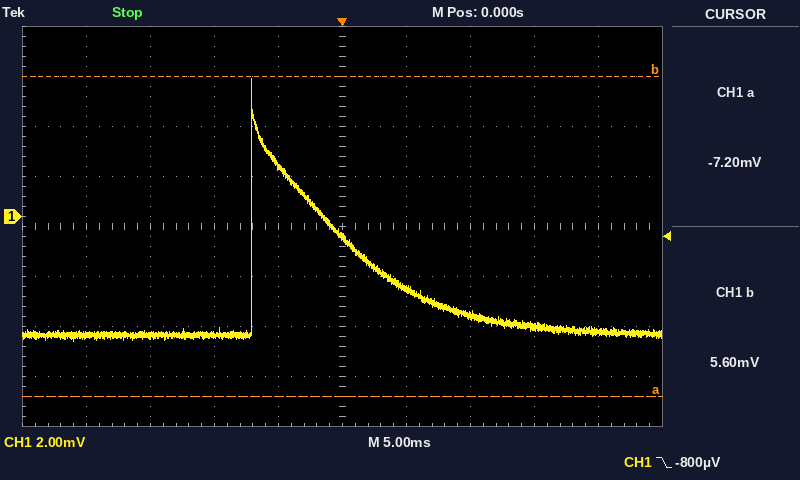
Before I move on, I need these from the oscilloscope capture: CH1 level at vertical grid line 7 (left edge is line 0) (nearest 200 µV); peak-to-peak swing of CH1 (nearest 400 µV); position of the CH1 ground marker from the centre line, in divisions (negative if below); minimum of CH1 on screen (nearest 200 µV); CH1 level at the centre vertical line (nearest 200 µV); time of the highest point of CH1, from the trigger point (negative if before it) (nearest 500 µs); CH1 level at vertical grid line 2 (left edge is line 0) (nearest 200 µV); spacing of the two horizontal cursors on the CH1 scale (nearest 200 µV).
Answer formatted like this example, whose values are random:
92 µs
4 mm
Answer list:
-4.0 mV
10.4 mV
+0.2 div
-5.0 mV
-800 µV
-7.0 ms
-4.8 mV
12.8 mV
